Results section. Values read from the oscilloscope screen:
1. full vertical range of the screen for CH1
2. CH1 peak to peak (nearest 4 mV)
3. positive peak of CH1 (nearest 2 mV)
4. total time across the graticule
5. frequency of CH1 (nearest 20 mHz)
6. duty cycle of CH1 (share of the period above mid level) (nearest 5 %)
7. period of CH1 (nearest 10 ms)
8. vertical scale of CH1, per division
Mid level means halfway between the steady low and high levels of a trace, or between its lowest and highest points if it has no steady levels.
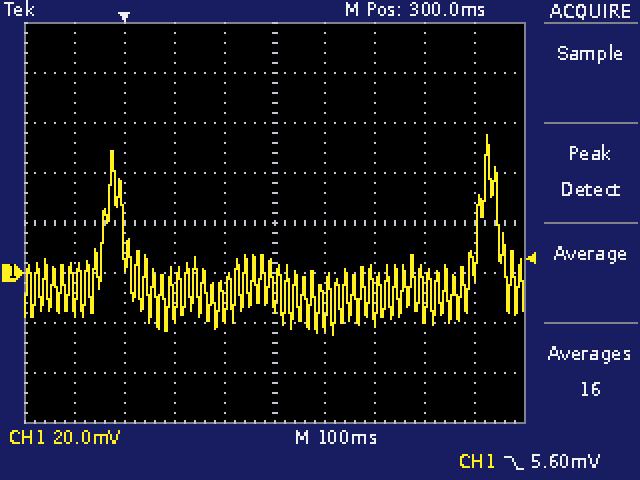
160 mV
80 mV
56 mV
1 s
1.34 Hz
5 %
750 ms
20 mV
